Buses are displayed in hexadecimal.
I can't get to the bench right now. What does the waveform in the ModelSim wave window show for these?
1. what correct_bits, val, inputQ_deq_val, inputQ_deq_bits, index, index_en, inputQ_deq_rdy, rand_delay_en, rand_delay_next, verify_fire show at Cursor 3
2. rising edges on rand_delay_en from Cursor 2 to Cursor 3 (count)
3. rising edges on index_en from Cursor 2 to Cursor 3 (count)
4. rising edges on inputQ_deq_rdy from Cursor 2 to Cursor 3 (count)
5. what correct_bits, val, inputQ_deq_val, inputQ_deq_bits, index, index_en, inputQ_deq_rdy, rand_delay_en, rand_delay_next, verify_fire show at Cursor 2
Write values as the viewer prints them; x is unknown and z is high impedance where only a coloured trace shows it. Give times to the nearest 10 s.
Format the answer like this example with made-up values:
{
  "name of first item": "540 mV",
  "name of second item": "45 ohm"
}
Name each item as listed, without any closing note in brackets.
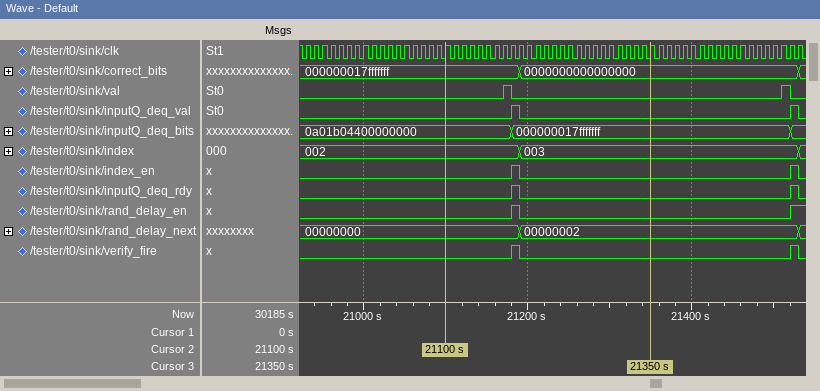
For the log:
{
  "what correct_bits, val, inputQ_deq_val, inputQ_deq_bits, index, index_en, inputQ_deq_rdy, rand_delay_en, rand_delay_next, verify_fire show at Cursor 3": "correct_bits=0000000000000000, val=0, inputQ_deq_val=0, inputQ_deq_bits=000000017fffffff, index=003, index_en=0, inputQ_deq_rdy=0, rand_delay_en=0, rand_delay_next=00000002, verify_fire=0",
  "rising edges on rand_delay_en from Cursor 2 to Cursor 3": "1",
  "rising edges on index_en from Cursor 2 to Cursor 3": "1",
  "rising edges on inputQ_deq_rdy from Cursor 2 to Cursor 3": "1",
  "what correct_bits, val, inputQ_deq_val, inputQ_deq_bits, index, index_en, inputQ_deq_rdy, rand_delay_en, rand_delay_next, verify_fire show at Cursor 2": "correct_bits=000000017fffffff, val=0, inputQ_deq_val=0, inputQ_deq_bits=0a01b04400000000, index=002, index_en=0, inputQ_deq_rdy=0, rand_delay_en=0, rand_delay_next=00000000, verify_fire=0"
}
